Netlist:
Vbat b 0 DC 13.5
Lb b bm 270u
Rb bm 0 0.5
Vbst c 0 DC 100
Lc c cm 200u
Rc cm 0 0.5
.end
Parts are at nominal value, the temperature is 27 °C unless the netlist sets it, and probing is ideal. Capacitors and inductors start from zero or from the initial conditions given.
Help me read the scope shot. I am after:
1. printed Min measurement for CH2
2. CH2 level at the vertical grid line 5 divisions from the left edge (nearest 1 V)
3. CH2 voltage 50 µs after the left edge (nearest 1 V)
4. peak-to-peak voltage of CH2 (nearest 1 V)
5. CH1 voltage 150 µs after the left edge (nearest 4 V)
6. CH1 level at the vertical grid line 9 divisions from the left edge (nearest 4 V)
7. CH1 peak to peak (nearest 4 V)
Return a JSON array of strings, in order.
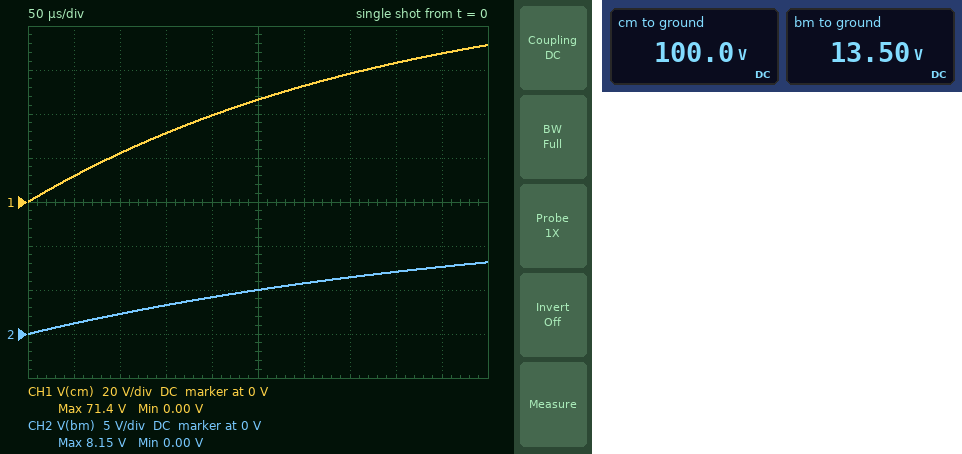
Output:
["0.00 V", "5 V", "1 V", "8 V", "32 V", "68 V", "72 V"]
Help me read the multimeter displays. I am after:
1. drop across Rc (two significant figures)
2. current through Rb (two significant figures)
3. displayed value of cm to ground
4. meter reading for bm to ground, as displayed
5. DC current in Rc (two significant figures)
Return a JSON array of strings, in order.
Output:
["100 V", "27 A", "100.0 V", "13.50 V", "200 A"]
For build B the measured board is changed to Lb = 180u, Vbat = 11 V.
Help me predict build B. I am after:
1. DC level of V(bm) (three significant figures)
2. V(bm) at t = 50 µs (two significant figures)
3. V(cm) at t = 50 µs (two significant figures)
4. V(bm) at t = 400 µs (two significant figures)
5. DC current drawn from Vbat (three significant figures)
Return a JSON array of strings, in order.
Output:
["11.0 V", "1.4 V", "12 V", "7.4 V", "22.0 A"]
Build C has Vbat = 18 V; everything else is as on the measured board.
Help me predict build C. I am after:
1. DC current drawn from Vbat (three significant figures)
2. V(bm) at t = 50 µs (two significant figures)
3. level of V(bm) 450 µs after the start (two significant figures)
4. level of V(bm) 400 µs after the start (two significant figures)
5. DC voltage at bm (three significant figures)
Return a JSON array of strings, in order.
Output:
["36.0 A", "1.6 V", "10 V", "9.4 V", "18.0 V"]
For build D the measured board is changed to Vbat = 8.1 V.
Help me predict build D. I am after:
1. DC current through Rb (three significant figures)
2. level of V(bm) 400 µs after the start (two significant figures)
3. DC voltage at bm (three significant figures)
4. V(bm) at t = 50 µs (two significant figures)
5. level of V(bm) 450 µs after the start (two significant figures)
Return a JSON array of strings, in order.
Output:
["16.2 A", "4.2 V", "8.10 V", "720 mV", "4.6 V"]
